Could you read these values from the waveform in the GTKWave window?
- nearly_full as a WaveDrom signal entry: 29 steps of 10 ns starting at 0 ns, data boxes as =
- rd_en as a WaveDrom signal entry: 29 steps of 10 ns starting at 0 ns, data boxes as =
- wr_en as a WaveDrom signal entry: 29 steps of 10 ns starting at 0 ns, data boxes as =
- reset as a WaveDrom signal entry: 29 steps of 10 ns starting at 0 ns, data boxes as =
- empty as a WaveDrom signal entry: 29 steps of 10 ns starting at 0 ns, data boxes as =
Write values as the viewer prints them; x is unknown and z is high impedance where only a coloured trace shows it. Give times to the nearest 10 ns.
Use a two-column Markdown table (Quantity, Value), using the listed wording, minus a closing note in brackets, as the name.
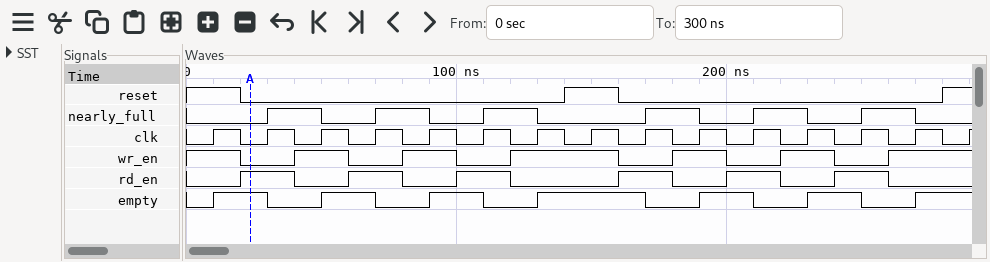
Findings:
| Quantity | Value |
|---|---|
| nearly_full as a WaveDrom signal entry: 29 steps of 10 ns starting at 0 ns, data boxes as = | {name: 'nearly_full', wave: '0..1.0.1.0.1.0...1.0.1.0.1.0.'} |
| rd_en as a WaveDrom signal entry: 29 steps of 10 ns starting at 0 ns, data boxes as = | {name: 'rd_en', wave: '0.1.0.1.0.1.0...1.0.1.0.1.0..'} |
| wr_en as a WaveDrom signal entry: 29 steps of 10 ns starting at 0 ns, data boxes as = | {name: 'wr_en', wave: '1.0.1.0.1.0.1...0.1.0.1.0.1..'} |
| reset as a WaveDrom signal entry: 29 steps of 10 ns starting at 0 ns, data boxes as = | {name: 'reset', wave: '1.0...........1.0...........1'} |
| empty as a WaveDrom signal entry: 29 steps of 10 ns starting at 0 ns, data boxes as = | {name: 'empty', wave: '01.0.1.0.1.0.1...0.1.0.1.0.1.'} |
